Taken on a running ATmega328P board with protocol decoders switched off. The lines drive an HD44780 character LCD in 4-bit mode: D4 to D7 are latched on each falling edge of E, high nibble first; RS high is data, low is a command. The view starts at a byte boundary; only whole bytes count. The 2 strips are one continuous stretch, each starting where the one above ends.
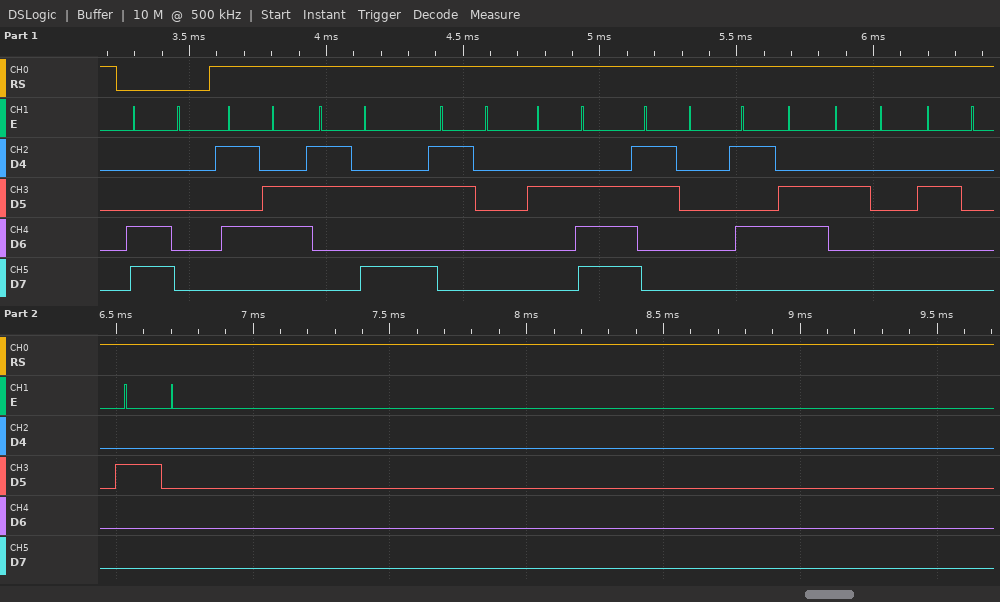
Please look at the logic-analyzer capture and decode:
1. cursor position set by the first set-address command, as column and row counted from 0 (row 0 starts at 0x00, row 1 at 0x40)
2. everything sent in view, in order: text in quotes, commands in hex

column 0, row 1
0xC0 "V:0.0V   "
